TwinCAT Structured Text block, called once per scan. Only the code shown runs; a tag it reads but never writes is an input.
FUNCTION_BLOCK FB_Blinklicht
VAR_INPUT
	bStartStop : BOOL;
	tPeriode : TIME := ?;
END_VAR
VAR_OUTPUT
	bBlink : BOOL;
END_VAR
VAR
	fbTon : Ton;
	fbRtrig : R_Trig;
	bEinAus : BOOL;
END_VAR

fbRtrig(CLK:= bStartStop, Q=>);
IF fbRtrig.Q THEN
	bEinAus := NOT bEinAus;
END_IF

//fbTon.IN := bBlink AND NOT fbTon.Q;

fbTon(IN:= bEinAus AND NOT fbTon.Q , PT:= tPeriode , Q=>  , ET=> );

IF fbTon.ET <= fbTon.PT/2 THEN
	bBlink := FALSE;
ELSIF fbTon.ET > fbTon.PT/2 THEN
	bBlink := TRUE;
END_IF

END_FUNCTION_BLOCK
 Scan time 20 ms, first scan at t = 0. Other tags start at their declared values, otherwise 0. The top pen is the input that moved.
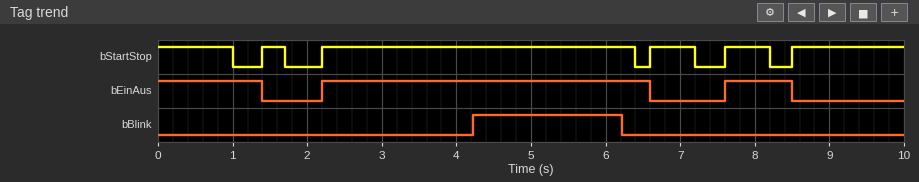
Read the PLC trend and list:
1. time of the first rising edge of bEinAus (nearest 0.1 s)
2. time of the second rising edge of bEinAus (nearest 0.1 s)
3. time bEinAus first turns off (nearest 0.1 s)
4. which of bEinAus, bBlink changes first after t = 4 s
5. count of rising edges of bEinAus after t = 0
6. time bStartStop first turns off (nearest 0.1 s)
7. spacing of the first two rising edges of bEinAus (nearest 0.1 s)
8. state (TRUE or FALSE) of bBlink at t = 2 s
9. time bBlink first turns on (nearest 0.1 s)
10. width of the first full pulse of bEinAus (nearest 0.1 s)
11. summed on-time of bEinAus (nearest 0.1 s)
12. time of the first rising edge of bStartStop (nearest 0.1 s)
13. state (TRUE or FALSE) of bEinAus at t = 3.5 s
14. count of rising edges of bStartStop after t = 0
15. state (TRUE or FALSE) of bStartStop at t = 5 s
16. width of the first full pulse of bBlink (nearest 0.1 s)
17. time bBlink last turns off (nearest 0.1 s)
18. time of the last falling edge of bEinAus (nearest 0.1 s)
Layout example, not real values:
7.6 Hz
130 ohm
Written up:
2.2 s
7.6 s
1.4 s
bBlink
2
1.0 s
5.4 s
FALSE
4.2 s
4.4 s
6.7 s
1.4 s
TRUE
5
TRUE
2.0 s
6.2 s
8.5 s
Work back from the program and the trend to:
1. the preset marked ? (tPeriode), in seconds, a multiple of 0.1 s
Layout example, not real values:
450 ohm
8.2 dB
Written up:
4.0 s
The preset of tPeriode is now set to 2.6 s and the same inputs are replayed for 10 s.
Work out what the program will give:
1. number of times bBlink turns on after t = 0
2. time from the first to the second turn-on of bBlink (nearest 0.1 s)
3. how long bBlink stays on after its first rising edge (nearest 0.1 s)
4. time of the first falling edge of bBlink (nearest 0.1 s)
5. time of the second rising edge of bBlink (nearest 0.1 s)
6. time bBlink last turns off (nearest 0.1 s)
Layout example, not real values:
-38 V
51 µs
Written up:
3
2.2 s
0.1 s
1.4 s
3.5 s
6.6 s
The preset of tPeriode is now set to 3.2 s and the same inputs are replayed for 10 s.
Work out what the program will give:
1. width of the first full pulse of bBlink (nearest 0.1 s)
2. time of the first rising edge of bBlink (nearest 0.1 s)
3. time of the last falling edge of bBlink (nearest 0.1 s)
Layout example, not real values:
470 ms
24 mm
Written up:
1.6 s
3.8 s
5.4 s
